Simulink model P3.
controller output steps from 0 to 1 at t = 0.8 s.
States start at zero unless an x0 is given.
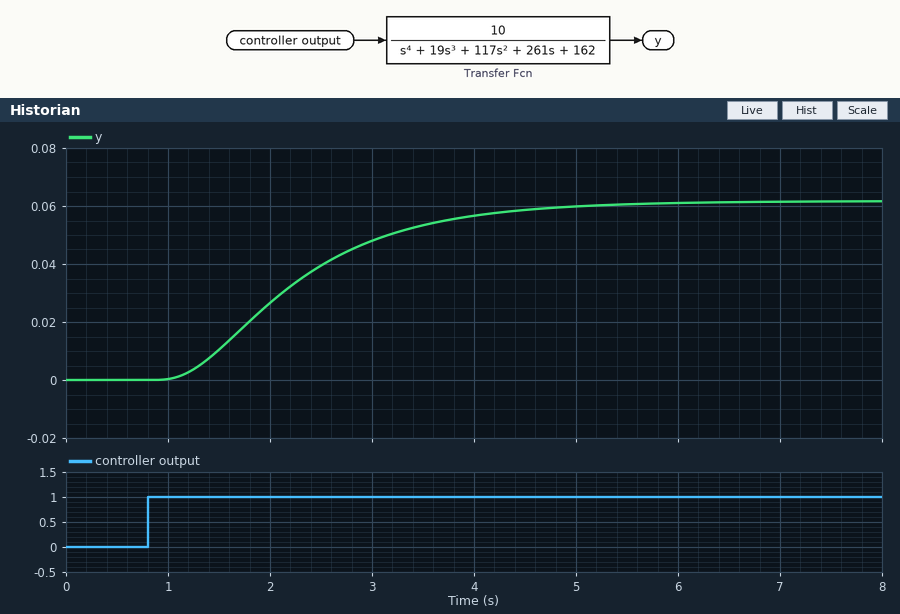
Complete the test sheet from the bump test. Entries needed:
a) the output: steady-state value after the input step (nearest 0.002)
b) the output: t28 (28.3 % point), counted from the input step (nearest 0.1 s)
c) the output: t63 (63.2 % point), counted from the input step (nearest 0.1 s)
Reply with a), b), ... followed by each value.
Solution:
a) 0.062
b) 0.9 s
c) 1.7 s
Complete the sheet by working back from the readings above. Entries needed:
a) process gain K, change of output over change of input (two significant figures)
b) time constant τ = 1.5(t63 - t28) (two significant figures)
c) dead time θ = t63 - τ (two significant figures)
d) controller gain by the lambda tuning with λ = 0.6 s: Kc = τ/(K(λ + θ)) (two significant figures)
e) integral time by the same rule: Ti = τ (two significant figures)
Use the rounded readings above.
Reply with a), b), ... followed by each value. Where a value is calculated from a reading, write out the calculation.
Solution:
a) (0.062 - 0) / 1 = 0.062
b) 1.5 × (1.7 - 0.9) = 1.2 s
c) 1.7 - 1.2 = 0.50 s
d) 1.2 / (0.062 × (0.6 + 0.5)) = 18
e) 1.2 s
